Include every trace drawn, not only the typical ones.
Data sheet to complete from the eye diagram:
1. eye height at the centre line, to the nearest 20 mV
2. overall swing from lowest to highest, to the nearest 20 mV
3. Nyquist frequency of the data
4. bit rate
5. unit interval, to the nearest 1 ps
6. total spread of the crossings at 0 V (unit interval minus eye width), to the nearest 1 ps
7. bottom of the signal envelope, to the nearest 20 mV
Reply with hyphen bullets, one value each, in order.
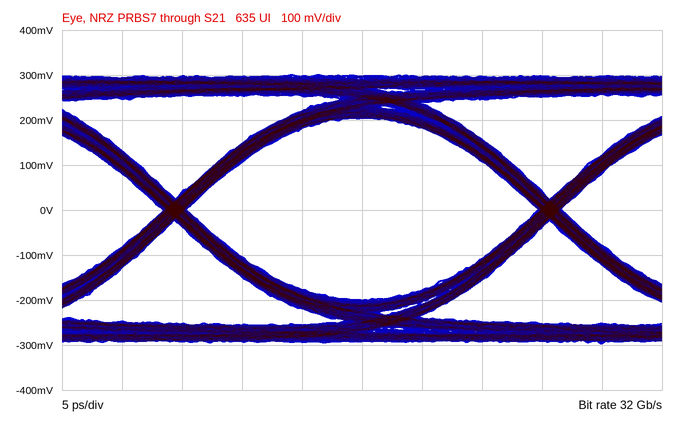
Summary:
- 400 mV
- 600 mV
- 16 GHz
- 32 Gb/s
- 31 ps
- 2 ps
- -300 mV
